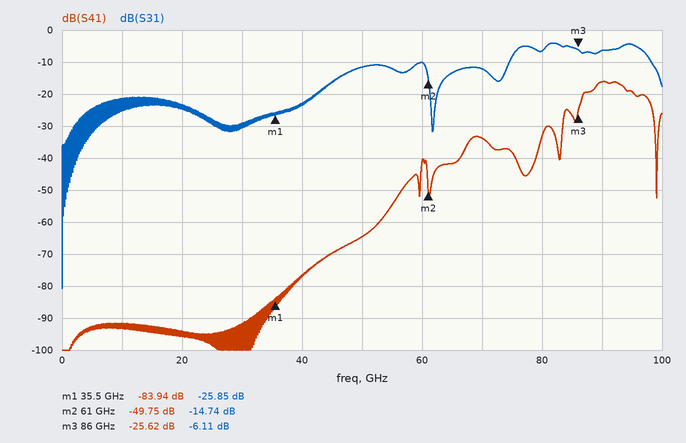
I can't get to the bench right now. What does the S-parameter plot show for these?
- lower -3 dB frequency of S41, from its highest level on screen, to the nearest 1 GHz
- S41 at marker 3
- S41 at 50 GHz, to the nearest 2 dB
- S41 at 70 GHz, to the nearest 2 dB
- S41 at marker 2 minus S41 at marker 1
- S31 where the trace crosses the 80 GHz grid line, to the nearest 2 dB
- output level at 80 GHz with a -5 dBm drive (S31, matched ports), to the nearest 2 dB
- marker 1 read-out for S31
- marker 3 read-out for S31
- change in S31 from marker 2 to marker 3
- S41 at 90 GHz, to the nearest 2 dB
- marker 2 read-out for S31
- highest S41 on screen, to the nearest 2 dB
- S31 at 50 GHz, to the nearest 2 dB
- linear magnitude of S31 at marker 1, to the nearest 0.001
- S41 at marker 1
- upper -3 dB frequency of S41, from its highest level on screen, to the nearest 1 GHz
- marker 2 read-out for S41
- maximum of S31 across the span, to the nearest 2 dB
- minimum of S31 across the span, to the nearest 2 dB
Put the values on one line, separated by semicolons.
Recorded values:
88 GHz; -25.62 dB; -64 dB; -34 dB; 34.19 dB; -6 dB; -12 dBm; -25.85 dB; -6.11 dB; 8.63 dB; -16 dB; -14.74 dB; -16 dB; -12 dB; 0.051; -83.94 dB; 95 GHz; -49.75 dB; -4 dB; -80 dB
